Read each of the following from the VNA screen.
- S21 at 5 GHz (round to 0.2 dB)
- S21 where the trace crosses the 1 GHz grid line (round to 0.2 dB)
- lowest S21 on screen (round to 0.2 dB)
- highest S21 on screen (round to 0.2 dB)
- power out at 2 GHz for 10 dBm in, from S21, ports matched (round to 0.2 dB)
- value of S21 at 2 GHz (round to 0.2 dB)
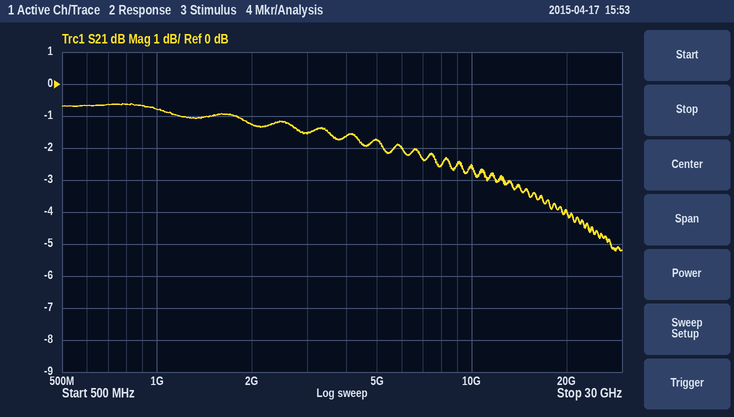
-1.8 dB
-0.8 dB
-5.2 dB
-0.6 dB
8.8 dBm
-1.2 dB
